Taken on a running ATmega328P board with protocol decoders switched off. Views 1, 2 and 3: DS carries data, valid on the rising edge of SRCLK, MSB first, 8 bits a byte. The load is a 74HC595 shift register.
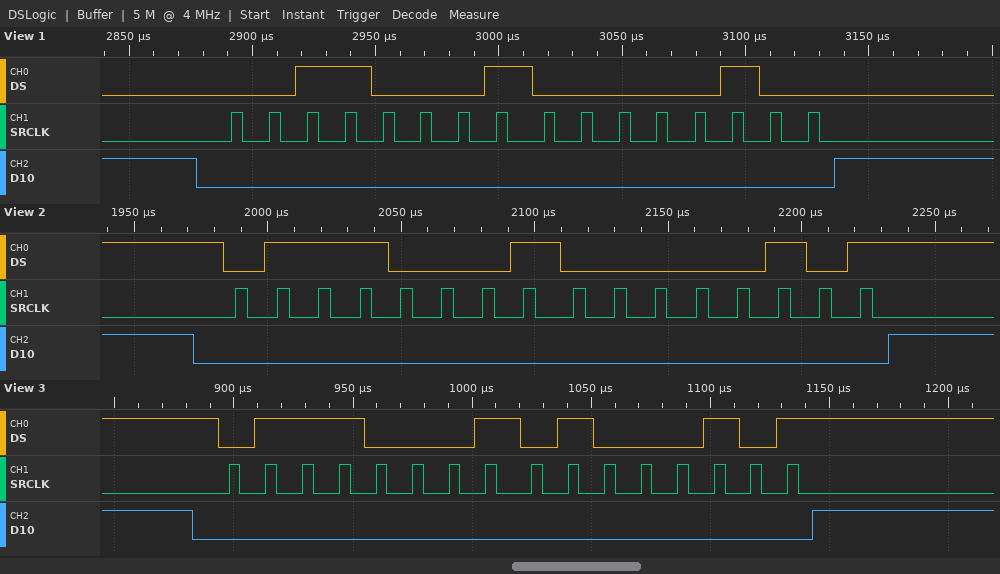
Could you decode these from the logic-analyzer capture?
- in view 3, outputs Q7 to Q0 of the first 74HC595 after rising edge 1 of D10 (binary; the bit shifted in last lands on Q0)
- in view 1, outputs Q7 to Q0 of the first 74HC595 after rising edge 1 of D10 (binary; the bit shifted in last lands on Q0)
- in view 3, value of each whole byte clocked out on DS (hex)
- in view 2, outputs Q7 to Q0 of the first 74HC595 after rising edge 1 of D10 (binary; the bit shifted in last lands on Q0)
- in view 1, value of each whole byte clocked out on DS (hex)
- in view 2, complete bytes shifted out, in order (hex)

01000101
00000100
0x71 0x45
00000101
0x31 0x04
71 05
